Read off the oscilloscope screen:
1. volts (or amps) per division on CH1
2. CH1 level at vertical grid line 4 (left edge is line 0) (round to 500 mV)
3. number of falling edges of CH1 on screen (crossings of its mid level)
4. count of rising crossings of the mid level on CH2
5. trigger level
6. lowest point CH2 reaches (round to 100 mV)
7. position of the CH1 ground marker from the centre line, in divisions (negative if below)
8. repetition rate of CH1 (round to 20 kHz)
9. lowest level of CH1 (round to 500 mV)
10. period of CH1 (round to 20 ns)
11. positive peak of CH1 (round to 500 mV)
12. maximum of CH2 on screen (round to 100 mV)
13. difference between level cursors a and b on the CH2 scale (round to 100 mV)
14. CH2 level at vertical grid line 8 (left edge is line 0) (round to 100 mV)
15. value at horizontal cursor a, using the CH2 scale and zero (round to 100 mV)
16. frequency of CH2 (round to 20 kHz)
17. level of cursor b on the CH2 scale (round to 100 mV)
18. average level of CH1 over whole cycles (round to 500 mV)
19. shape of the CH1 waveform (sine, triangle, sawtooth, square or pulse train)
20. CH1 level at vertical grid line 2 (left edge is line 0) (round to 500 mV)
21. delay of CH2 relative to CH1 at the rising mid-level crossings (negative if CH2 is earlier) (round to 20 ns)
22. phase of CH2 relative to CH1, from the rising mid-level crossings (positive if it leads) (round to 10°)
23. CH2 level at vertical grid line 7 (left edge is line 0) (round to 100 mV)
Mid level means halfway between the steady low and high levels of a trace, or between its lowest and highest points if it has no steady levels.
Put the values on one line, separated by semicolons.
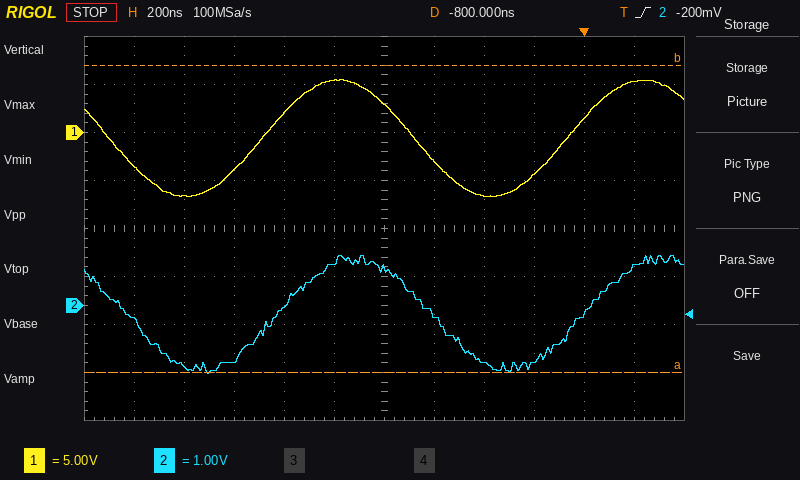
5 V; 2.0 V; 2; 2; -200 mV; -1.4 V; +2.0 div; 820 kHz; -6.5 V; 1.22 µs; 5.5 V; 1.0 V; 6.4 V; -1.2 V; -1.4 V; 820 kHz; 5.0 V; -500 mV; sine; -6.5 V; +60 ns; -20°; -200 mV
